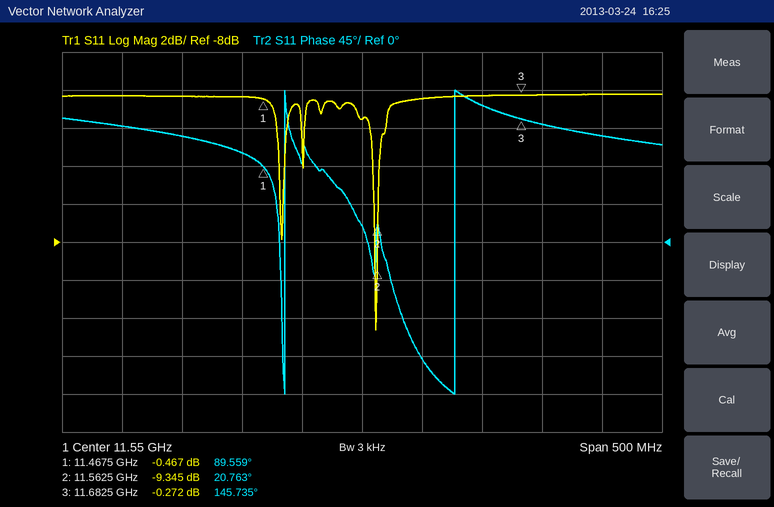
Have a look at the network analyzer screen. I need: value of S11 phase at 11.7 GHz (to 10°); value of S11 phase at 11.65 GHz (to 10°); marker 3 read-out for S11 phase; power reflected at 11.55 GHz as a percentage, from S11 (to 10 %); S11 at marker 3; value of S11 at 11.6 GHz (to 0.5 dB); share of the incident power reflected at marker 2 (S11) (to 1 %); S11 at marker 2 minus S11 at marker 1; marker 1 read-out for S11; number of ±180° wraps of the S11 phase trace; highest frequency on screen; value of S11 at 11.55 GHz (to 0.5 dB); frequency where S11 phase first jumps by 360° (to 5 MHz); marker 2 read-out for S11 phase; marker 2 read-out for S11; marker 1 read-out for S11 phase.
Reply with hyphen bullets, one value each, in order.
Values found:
- 140°
- 160°
- 145.735°
- 70 %
- -0.272 dB
- -0.5 dB
- 12 %
- -8.878 dB
- -0.467 dB
- 2
- 11.8 GHz
- -1.5 dB
- 11.485 GHz
- 20.763°
- -9.345 dB
- 89.559°
